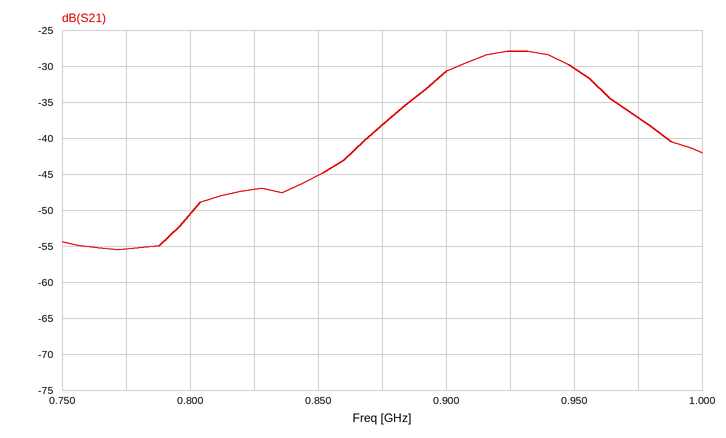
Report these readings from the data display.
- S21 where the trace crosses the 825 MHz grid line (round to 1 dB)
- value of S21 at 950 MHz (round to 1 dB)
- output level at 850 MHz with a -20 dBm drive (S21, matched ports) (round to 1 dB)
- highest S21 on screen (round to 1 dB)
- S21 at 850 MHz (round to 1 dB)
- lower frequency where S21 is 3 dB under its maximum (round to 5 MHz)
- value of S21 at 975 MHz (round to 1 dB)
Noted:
-47 dB
-30 dB
-65 dBm
-28 dB
-45 dB
900 MHz
-37 dB
